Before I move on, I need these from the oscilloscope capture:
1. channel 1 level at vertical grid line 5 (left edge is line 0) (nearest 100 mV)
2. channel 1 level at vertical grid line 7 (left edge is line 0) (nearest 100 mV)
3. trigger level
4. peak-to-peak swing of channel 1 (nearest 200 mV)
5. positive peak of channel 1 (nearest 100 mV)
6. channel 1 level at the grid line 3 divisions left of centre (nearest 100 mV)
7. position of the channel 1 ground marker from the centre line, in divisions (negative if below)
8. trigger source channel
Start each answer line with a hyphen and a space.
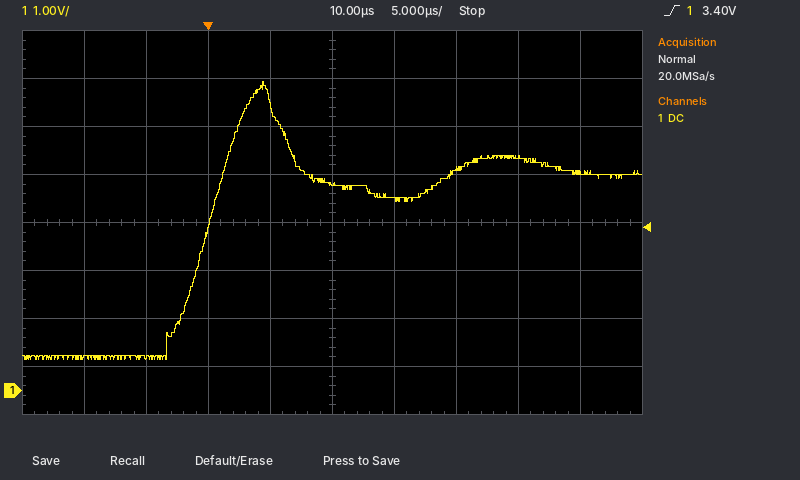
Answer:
- 4.3 V
- 4.6 V
- 3.40 V
- 5.8 V
- 6.4 V
- 700 mV
- -3.5 div
- channel 1
